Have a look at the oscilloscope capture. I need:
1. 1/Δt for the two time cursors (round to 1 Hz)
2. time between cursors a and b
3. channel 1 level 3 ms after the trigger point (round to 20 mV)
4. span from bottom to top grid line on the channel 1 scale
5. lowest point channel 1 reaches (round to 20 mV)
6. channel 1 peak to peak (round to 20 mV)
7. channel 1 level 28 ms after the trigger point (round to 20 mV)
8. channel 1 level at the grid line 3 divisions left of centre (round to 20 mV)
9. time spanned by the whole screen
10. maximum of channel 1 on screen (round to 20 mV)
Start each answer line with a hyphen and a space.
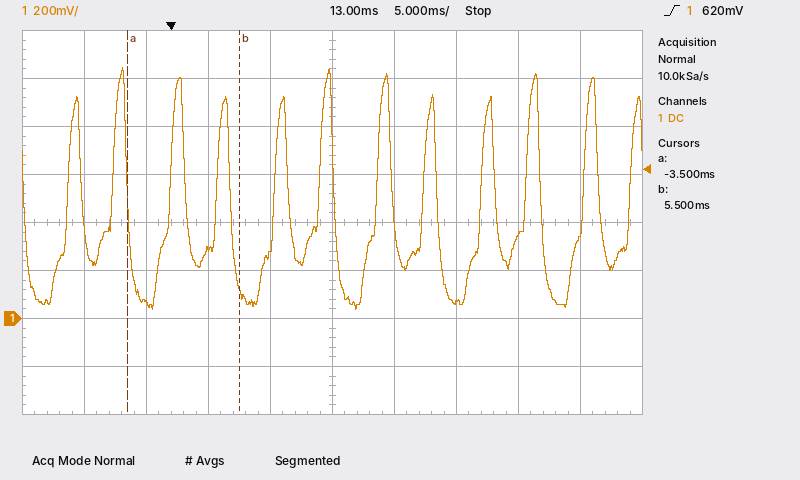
- 111 Hz
- 9.0 ms
- 280 mV
- 1.6 V
- 40 mV
- 1.00 V
- 340 mV
- 60 mV
- 50 ms
- 1.04 V
